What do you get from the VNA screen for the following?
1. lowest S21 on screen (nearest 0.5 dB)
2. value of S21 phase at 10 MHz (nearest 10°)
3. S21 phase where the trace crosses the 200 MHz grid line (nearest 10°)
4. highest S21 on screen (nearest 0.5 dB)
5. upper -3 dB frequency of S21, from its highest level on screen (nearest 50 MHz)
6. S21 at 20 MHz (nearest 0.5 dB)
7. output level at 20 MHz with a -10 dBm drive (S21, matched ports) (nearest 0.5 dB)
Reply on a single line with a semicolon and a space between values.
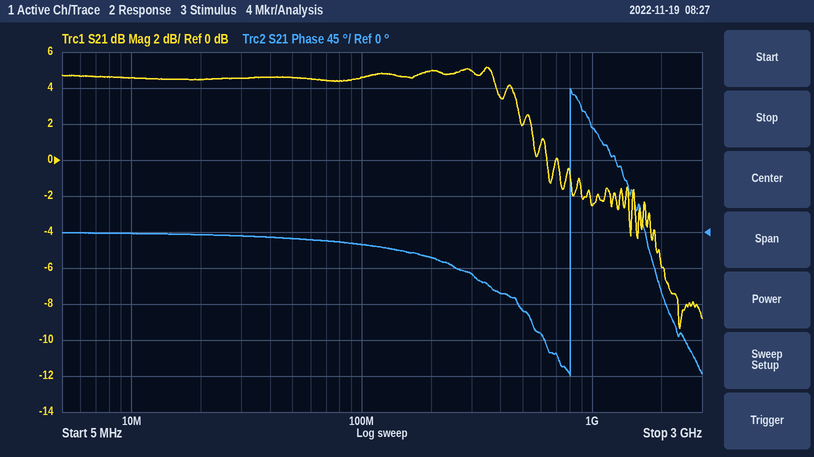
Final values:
-9.5 dB; 0°; -30°; 5.0 dB; 500 MHz; 4.5 dB; -5.5 dBm
